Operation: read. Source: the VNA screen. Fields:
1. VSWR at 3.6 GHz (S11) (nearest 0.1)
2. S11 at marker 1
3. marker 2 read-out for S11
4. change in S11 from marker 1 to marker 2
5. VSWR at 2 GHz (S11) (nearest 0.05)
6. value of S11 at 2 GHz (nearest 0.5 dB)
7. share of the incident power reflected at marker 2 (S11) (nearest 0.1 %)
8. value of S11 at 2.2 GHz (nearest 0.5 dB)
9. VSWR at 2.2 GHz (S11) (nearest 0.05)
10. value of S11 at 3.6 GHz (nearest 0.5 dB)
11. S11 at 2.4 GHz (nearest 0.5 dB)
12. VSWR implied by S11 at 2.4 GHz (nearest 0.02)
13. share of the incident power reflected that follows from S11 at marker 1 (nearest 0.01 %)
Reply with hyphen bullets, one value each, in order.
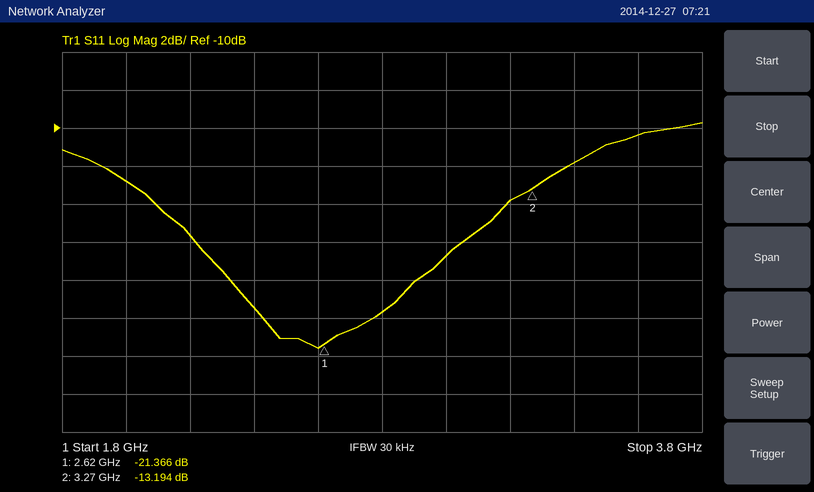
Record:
- 1.9
- -21.366 dB
- -13.194 dB
- 8.172 dB
- 1.60
- -13.0 dB
- 4.8 %
- -15.5 dB
- 1.40
- -10.5 dB
- -19.5 dB
- 1.24
- 0.73 %
